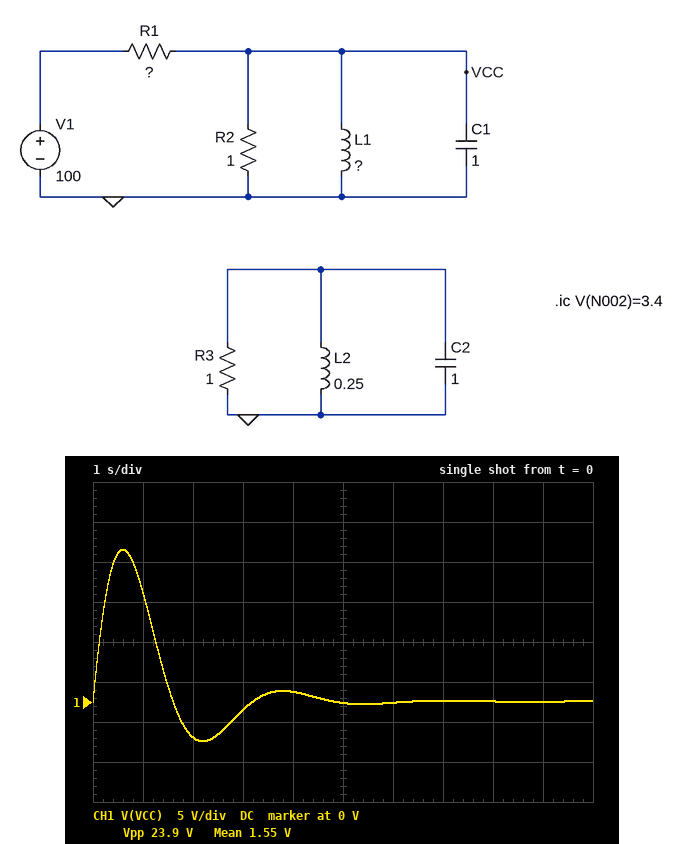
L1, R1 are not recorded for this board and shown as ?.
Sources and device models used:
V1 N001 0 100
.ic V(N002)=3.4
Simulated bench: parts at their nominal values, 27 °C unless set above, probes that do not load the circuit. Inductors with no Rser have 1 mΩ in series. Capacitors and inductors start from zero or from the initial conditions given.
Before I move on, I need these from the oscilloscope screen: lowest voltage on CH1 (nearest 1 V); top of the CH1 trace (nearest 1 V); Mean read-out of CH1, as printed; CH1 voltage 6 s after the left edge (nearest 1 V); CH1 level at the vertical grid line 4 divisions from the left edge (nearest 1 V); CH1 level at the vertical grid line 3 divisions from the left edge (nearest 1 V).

-5 V
19 V
1.55 V
0 V
1 V
-1 V
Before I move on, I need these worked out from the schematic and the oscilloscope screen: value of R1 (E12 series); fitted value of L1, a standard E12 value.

1.5 Ω
220 mH
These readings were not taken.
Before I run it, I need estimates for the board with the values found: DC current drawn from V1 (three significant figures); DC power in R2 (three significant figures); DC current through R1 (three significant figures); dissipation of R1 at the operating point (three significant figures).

66.6 A
4.43 mW
66.6 A
6.66 kW
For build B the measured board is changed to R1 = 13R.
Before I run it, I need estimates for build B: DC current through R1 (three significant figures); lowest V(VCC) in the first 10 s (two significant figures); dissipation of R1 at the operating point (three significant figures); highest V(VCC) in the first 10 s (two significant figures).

7.69 A
-1.1 V
769 W
2.6 V
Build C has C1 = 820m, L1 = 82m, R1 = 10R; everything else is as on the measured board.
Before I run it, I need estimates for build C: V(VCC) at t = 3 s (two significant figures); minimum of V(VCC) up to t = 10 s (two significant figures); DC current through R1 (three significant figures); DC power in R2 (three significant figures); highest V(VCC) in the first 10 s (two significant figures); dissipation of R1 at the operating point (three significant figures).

-380 mV
-1.4 V
10.0 A
99.8 µW
2.5 V
1.00 kW
